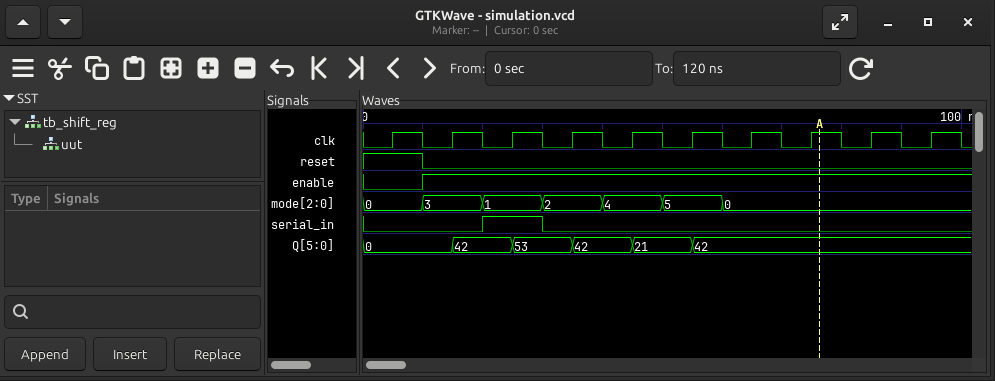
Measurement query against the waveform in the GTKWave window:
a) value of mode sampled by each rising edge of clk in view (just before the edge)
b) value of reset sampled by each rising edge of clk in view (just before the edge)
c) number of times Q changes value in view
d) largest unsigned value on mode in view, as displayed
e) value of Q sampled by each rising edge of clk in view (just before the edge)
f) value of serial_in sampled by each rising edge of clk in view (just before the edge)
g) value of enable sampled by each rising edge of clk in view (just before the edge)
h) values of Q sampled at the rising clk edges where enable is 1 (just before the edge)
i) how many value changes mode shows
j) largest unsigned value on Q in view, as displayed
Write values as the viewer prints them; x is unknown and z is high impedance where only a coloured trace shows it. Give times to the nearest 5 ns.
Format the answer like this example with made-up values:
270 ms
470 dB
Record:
0, 3, 1, 2, 4, 5, 0, 0, 0, 0
1 0 0 0 0 0 0 0 0 0
5
5
0, 0, 42, 53, 42, 21, 42, 42, 42, 42
0 0 1 0 0 0 0 0 0 0
0 1 1 1 1 1 1 1 1 1
0, 42, 53, 42, 21, 42, 42, 42, 42
6
53
